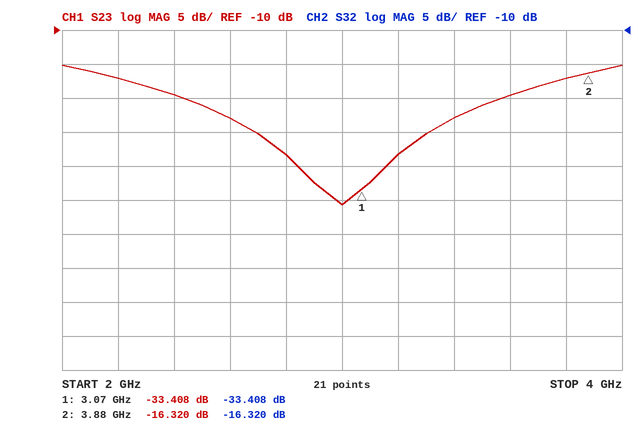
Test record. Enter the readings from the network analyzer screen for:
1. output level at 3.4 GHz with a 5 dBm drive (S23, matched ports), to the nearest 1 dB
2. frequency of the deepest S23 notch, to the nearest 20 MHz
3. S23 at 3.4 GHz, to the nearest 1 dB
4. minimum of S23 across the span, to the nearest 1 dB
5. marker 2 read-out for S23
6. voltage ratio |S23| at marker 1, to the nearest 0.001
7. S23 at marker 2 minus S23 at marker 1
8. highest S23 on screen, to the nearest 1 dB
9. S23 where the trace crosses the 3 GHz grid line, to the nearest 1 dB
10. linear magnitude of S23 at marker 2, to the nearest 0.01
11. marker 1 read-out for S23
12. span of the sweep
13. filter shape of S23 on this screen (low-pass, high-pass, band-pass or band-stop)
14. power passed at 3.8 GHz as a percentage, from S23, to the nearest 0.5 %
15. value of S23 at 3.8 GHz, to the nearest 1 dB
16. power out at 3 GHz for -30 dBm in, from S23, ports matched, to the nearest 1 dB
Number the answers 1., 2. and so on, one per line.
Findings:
1. -18 dBm
2. 3.00 GHz
3. -23 dB
4. -36 dB
5. -16.320 dB
6. 0.021
7. 17.088 dB
8. -15 dB
9. -36 dB
10. 0.15
11. -33.408 dB
12. 2 GHz
13. band-stop
14. 2.0 %
15. -17 dB
16. -66 dBm
